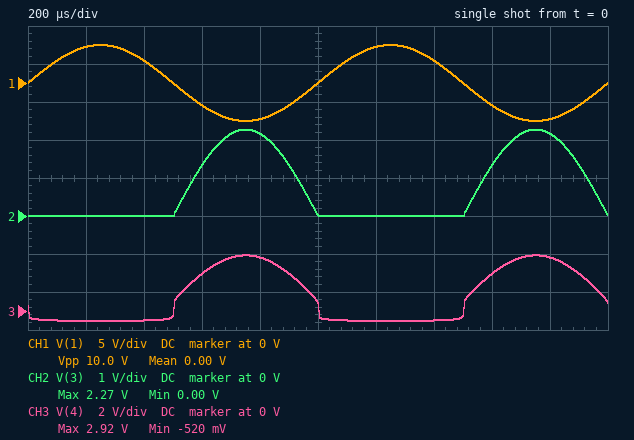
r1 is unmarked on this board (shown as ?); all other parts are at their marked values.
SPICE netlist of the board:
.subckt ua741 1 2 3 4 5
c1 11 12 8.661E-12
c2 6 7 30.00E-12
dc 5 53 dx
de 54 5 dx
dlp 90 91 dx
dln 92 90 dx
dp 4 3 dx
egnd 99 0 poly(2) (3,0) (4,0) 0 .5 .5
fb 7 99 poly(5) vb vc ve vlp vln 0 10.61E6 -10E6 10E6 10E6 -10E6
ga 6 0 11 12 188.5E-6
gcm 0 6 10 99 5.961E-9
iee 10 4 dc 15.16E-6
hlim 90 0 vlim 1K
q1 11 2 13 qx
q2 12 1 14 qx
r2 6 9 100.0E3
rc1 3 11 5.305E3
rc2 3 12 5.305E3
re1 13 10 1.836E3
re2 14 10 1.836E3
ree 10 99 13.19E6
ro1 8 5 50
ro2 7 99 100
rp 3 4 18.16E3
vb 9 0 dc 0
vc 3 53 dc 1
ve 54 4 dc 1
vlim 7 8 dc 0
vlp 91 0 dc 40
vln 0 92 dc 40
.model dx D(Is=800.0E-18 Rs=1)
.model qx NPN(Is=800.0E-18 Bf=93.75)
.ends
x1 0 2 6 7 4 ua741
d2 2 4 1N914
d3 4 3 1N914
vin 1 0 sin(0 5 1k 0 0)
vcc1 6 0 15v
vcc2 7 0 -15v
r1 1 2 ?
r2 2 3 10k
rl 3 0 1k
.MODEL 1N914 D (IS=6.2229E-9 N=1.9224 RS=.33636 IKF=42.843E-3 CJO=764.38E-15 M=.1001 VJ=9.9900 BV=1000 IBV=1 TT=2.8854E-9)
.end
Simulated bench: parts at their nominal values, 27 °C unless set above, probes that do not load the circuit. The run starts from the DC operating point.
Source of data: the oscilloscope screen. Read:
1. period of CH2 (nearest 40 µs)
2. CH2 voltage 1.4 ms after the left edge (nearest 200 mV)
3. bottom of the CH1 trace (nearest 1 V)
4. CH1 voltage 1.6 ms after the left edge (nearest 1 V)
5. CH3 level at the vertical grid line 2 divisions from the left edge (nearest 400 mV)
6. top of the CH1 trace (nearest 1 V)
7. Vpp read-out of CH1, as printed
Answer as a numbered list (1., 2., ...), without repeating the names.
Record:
1. 1.00 ms
2. 0 V
3. -5 V
4. -3 V
5. -400 mV
6. 5 V
7. 10.0 V
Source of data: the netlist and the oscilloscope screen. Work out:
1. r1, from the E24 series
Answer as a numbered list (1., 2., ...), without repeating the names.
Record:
1. 22 kΩ
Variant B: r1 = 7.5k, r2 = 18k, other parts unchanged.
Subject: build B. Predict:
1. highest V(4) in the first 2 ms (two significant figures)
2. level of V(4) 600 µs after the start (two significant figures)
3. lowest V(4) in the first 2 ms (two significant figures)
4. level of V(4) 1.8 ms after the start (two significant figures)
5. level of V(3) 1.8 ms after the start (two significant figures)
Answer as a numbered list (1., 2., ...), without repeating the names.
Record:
1. 13 V
2. 7.7 V
3. -580 mV
4. 12 V
5. 11 V
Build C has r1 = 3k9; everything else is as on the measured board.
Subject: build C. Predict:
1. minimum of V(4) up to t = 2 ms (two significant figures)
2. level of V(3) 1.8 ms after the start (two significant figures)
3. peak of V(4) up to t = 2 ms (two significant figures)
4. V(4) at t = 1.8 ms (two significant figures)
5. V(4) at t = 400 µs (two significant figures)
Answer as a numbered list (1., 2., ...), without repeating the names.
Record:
1. -620 mV
2. 12 V
3. 14 V
4. 13 V
5. -590 mV
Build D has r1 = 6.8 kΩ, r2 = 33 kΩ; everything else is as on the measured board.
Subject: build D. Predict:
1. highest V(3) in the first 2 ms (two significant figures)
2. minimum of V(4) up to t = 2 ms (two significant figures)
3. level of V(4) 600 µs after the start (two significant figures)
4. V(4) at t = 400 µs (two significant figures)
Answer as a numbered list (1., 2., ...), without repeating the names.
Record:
1. 14 V
2. -590 mV
3. 15 V
4. -560 mV
